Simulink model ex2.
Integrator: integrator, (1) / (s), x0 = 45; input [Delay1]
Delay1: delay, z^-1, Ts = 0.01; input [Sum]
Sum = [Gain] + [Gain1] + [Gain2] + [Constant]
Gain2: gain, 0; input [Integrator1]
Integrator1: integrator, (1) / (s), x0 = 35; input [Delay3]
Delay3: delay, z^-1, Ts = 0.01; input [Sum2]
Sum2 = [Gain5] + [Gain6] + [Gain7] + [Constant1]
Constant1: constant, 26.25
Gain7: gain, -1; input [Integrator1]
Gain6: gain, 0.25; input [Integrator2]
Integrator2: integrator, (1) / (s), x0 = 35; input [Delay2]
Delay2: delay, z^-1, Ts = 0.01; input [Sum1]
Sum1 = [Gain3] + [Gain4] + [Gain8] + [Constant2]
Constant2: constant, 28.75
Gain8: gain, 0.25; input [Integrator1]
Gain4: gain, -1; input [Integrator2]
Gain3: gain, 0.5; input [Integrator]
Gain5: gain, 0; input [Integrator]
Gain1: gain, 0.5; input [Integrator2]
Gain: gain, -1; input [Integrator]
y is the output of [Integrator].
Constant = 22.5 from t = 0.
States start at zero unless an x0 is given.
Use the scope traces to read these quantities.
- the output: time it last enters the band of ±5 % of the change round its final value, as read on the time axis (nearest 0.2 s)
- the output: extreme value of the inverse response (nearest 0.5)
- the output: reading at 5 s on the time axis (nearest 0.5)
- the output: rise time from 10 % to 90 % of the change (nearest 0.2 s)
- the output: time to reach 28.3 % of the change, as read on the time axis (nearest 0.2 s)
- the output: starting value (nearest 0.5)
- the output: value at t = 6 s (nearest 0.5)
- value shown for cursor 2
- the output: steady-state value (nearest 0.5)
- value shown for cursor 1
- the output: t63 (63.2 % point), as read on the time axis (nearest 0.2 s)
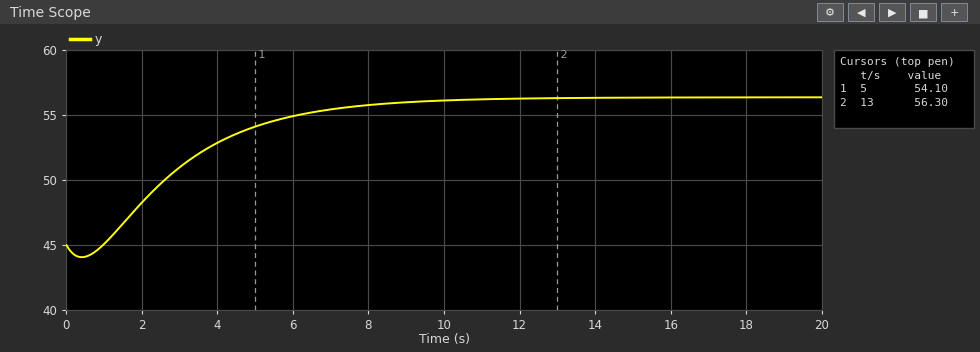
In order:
8.2 s
44.0
54.0
5.2 s
2.0 s
45.0
55.0
56.30
56.5
54.10
3.6 s
